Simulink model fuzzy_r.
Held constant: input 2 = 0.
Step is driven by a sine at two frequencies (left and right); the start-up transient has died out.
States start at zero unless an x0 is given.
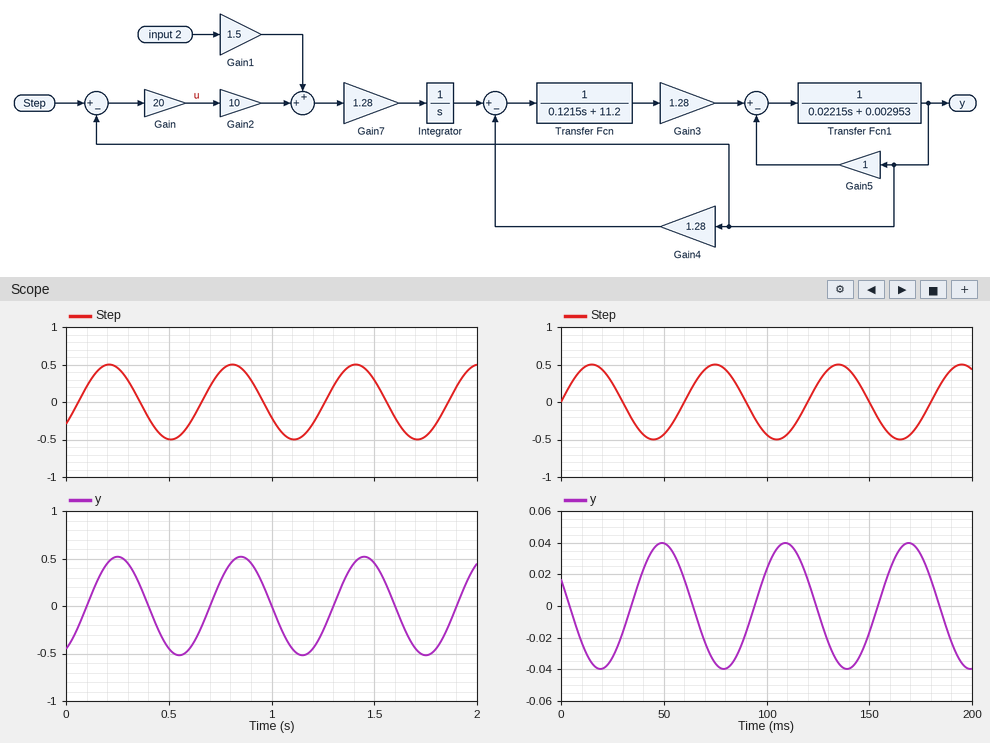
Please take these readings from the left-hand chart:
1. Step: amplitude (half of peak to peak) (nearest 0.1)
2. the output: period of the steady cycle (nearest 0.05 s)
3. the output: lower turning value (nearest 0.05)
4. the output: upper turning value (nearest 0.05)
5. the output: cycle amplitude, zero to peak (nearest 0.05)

0.5
0.60 s
-0.50
0.50
0.50
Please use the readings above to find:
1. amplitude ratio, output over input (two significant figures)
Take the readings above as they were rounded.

1.0
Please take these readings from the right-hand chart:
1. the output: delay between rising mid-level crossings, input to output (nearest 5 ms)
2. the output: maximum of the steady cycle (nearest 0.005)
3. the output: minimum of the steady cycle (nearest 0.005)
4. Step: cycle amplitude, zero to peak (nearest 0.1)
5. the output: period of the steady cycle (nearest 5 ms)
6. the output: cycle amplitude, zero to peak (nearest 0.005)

35 ms
0.040
-0.040
0.5
60 ms
0.040
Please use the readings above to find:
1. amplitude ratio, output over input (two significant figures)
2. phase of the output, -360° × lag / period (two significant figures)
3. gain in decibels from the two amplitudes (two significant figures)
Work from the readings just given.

0.080
-210°
-22 dB
